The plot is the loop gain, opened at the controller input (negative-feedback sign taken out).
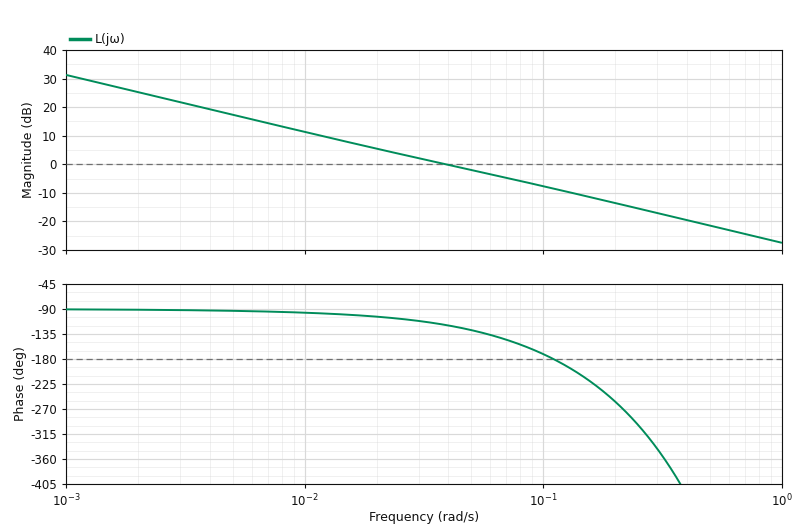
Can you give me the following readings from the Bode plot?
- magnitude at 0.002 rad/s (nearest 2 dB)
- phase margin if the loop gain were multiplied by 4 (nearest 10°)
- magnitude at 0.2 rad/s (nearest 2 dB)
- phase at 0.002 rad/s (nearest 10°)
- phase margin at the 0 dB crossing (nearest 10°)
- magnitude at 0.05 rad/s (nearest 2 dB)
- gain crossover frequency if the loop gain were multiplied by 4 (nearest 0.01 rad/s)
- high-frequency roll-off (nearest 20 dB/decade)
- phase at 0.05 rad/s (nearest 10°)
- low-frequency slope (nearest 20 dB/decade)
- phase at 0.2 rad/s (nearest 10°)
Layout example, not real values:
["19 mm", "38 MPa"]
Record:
["26 dB", "-50°", "-14 dB", "-90°", "60°", "-2 dB", "0.17 rad/s", "-20 dB/decade", "-130°", "-20 dB/decade", "-260°"]
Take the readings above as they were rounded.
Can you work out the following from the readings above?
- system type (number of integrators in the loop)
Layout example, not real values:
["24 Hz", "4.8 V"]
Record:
["1"]
